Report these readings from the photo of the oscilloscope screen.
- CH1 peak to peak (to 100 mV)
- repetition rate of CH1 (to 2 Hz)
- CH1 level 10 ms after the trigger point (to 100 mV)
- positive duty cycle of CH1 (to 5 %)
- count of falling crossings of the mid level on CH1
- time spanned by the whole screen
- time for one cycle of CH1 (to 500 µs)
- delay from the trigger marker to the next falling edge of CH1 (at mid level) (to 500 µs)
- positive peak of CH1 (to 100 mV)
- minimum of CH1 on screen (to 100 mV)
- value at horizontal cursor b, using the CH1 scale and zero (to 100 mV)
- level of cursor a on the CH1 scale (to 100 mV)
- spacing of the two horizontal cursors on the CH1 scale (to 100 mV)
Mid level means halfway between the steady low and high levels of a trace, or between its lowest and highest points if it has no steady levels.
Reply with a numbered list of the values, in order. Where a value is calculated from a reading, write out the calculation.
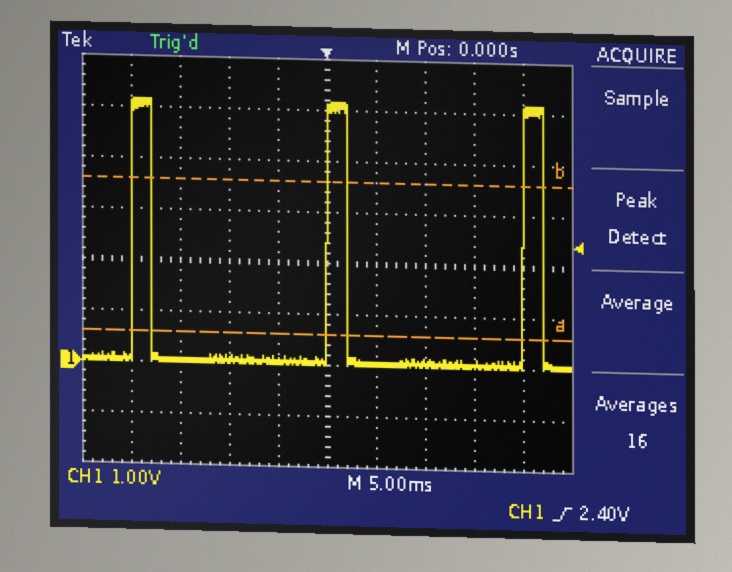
1. 5.2 V − (0.0 V) = 5.2 V
2. 1 / 20.0 ms ≈ 50 Hz
3. 100 mV
4. 10 %
5. 3
6. 50 ms
7. 20.0 ms
8. 2.0 ms
9. 5.2 V
10. 0.0 V
11. 3.6 V
12. 600 mV
13. 3.0 V
